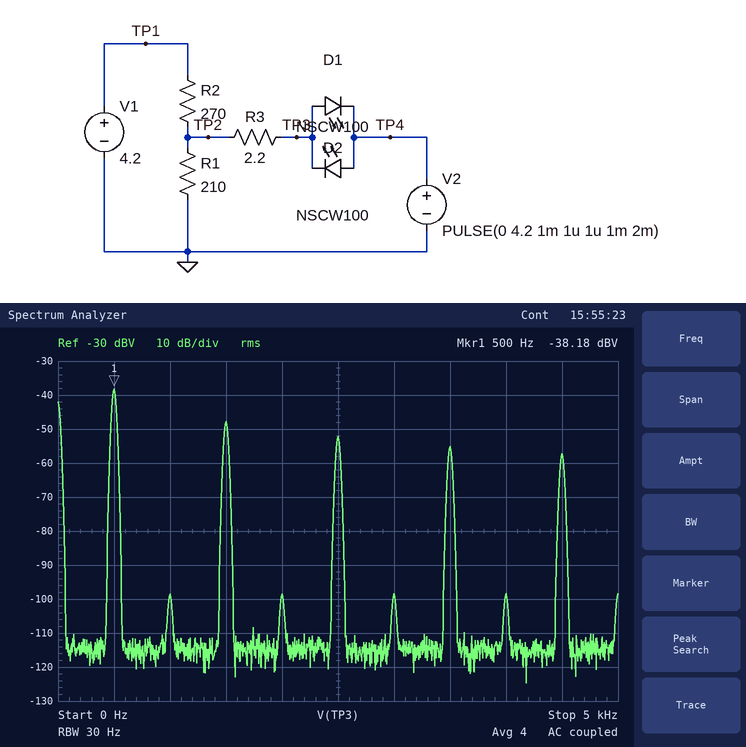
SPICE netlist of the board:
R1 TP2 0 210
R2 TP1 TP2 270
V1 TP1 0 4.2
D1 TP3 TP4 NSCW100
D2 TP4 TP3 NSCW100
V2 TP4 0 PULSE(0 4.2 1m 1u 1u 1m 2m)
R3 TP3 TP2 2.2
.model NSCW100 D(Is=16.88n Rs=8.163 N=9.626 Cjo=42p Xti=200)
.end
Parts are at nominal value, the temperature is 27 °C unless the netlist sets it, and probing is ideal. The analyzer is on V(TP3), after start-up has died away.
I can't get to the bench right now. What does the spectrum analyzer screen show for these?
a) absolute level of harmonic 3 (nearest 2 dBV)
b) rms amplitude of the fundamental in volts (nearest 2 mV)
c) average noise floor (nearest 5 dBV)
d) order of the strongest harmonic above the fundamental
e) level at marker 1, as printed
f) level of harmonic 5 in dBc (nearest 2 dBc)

-48 dBV
12 mV
-115 dBV
3
-38.18 dBV
-14 dBc
